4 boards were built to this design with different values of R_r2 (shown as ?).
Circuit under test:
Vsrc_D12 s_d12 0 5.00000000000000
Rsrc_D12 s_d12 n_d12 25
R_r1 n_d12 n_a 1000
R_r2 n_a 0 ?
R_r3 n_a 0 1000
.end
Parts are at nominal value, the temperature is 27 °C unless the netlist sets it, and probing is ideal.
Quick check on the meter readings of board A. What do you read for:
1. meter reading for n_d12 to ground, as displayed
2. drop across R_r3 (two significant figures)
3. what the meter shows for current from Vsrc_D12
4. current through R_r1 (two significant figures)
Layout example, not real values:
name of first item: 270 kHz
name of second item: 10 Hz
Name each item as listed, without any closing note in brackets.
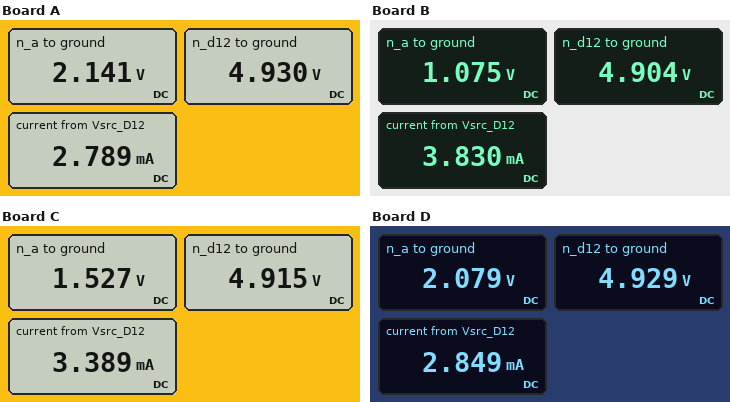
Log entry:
meter reading for n_d12 to ground, as displayed: 4.930 V
drop across R_r3: 2.1 V
what the meter shows for current from Vsrc_D12: 2.789 mA
current through R_r1: 2.8 mA
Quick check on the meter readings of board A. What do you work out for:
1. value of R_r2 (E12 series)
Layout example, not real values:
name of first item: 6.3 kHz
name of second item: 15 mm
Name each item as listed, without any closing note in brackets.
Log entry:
value of R_r2: 3.3 kΩ
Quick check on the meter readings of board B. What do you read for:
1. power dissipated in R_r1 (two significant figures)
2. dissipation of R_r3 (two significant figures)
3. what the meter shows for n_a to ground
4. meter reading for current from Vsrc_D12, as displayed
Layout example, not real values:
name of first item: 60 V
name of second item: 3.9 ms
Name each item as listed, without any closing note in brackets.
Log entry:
power dissipated in R_r1: 15 mW
dissipation of R_r3: 1.2 mW
what the meter shows for n_a to ground: 1.075 V
meter reading for current from Vsrc_D12, as displayed: 3.830 mA
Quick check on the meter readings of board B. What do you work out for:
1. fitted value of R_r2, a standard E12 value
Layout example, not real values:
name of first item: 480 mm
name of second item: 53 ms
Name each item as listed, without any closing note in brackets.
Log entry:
fitted value of R_r2, a standard E12 value: 390 Ω
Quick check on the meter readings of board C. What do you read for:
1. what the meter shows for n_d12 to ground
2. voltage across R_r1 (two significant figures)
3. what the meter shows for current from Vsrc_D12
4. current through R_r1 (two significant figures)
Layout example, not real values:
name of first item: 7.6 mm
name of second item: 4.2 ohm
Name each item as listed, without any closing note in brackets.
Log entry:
what the meter shows for n_d12 to ground: 4.915 V
voltage across R_r1: 3.4 V
what the meter shows for current from Vsrc_D12: 3.389 mA
current through R_r1: 3.4 mA
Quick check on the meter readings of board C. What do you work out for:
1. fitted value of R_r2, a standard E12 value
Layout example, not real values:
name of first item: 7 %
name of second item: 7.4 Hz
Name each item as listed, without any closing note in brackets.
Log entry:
fitted value of R_r2, a standard E12 value: 820 Ω
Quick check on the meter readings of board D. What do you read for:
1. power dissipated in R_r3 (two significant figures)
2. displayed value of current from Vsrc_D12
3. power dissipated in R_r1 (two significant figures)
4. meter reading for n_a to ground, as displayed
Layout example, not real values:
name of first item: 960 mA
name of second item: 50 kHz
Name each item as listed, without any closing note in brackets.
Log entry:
power dissipated in R_r3: 4.3 mW
displayed value of current from Vsrc_D12: 2.849 mA
power dissipated in R_r1: 8.1 mW
meter reading for n_a to ground, as displayed: 2.079 V
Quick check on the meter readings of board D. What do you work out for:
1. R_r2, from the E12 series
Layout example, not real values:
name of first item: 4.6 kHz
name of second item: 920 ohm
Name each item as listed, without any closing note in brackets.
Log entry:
R_r2, from the E12 series: 2.7 kΩ
